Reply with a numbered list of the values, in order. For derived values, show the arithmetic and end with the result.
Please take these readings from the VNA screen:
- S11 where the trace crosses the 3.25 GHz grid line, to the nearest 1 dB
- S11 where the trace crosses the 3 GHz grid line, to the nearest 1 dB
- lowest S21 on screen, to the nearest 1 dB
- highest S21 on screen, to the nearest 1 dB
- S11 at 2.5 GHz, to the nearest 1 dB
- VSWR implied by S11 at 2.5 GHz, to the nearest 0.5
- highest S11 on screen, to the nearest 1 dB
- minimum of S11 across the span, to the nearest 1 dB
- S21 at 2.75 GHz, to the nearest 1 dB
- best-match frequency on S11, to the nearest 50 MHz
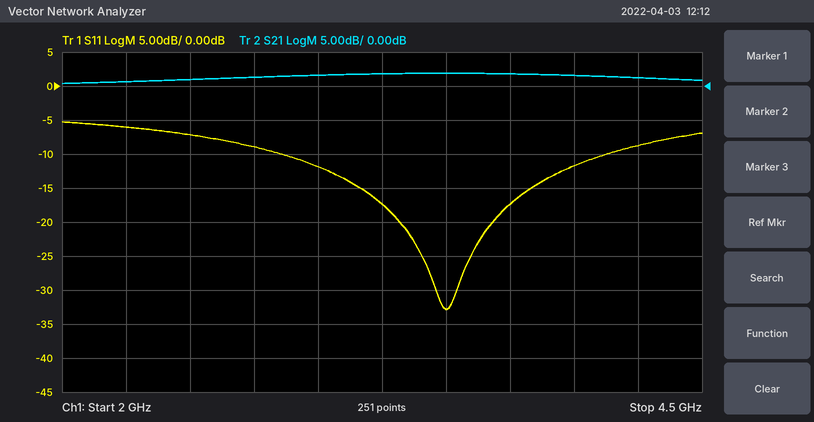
1. -17 dB
2. -12 dB
3. 0 dB
4. 2 dB
5. -7 dB
6. |Γ| = 10^(-7/20) = 0.4467; VSWR = (1 + 0.4467)/(1 − 0.4467) ≈ 2.61, so 2.5 to the nearest 0.5
7. -5 dB
8. -33 dB
9. 1 dB
10. 3.50 GHz
